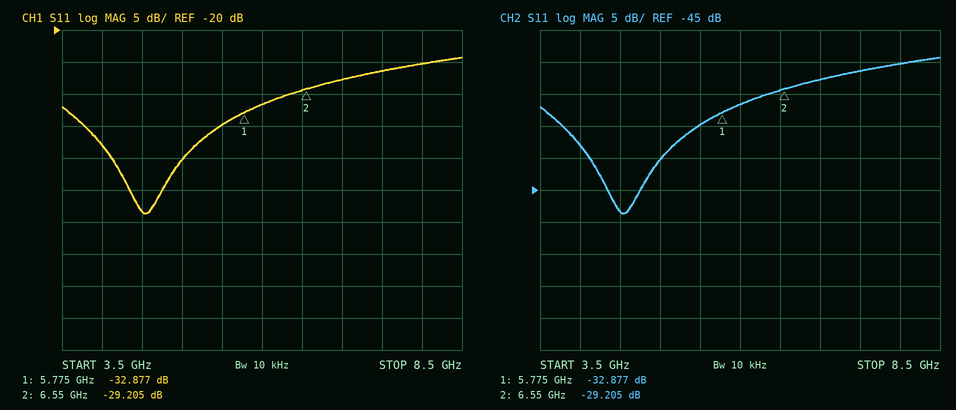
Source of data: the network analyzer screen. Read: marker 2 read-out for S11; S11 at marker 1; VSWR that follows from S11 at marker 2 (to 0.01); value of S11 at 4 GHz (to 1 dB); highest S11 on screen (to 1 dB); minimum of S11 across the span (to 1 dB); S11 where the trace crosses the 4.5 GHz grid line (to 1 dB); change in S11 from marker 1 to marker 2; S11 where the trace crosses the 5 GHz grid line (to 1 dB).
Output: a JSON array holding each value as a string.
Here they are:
["-29.205 dB", "-32.877 dB", "1.07", "-38 dB", "-24 dB", "-49 dB", "-48 dB", "3.672 dB", "-40 dB"]
